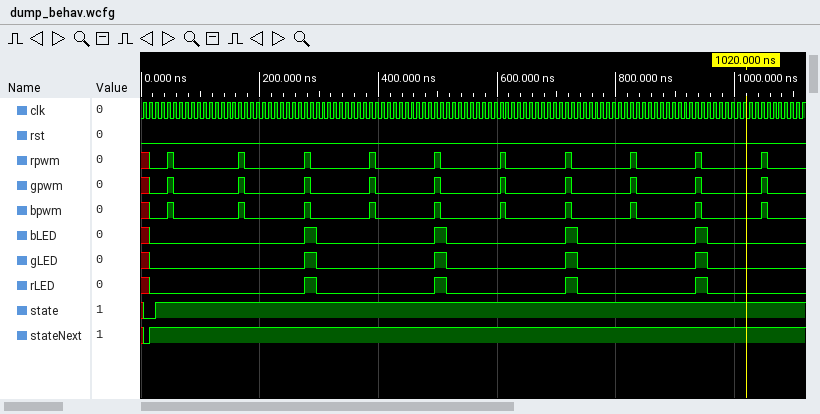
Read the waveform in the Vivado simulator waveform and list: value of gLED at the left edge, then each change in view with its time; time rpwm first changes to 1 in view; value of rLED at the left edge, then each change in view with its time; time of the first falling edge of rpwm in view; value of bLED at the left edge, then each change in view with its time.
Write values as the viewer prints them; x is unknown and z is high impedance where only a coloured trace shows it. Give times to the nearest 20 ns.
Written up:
x, 0 at 20 ns, 1 at 280 ns, 0 at 300 ns, 1 at 500 ns, 0 at 520 ns, 1 at 720 ns, 0 at 740 ns, 1 at 940 ns, 0 at 960 ns
40 ns
x, 0 at 20 ns, 1 at 280 ns, 0 at 300 ns, 1 at 500 ns, 0 at 520 ns, 1 at 720 ns, 0 at 740 ns, 1 at 940 ns, 0 at 960 ns
60 ns
x, 0 at 20 ns, 1 at 280 ns, 0 at 300 ns, 1 at 500 ns, 0 at 520 ns, 1 at 720 ns, 0 at 740 ns, 1 at 940 ns, 0 at 960 ns
